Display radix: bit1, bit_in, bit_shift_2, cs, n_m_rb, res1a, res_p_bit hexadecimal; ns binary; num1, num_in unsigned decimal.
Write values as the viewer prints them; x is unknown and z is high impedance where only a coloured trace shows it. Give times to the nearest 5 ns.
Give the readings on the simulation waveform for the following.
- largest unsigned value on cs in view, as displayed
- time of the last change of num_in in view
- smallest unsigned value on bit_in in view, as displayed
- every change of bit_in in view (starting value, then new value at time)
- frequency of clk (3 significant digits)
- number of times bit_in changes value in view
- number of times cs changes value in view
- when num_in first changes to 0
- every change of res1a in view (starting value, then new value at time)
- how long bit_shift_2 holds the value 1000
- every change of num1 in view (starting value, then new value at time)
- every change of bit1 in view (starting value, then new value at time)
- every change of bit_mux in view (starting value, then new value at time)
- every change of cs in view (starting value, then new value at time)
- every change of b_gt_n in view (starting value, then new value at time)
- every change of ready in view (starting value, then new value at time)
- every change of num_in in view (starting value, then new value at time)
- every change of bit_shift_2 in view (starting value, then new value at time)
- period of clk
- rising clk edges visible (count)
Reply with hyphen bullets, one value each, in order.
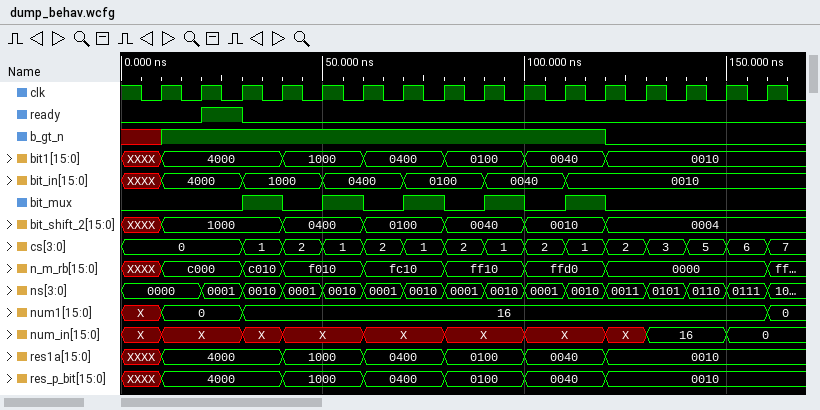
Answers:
- 7
- 150 ns
- 0010
- XXXX, 4000 at 10 ns, 1000 at 30 ns, 0400 at 50 ns, 0100 at 70 ns, 0040 at 90 ns, 0010 at 110 ns
- 100 MHz
- 6
- 14
- 150 ns
- XXXX, 4000 at 10 ns, 1000 at 40 ns, 0400 at 60 ns, 0100 at 80 ns, 0040 at 100 ns, 0010 at 120 ns
- 30 ns
- X, 0 at 10 ns, 16 at 30 ns, 0 at 160 ns
- XXXX, 4000 at 10 ns, 1000 at 40 ns, 0400 at 60 ns, 0100 at 80 ns, 0040 at 100 ns, 0010 at 120 ns
- 0, 1 at 30 ns, 0 at 40 ns, 1 at 50 ns, 0 at 60 ns, 1 at 70 ns, 0 at 80 ns, 1 at 90 ns, 0 at 100 ns, 1 at 110 ns, 0 at 120 ns
- 0, 1 at 30 ns, 2 at 40 ns, 1 at 50 ns, 2 at 60 ns, 1 at 70 ns, 2 at 80 ns, 1 at 90 ns, 2 at 100 ns, 1 at 110 ns, 2 at 120 ns, 3 at 130 ns, 5 at 140 ns, 6 at 150 ns, 7 at 160 ns
- x, 1 at 10 ns, 0 at 120 ns
- 0, 1 at 20 ns, 0 at 30 ns
- X, X at 10 ns, X at 30 ns, X at 40 ns, X at 60 ns, X at 80 ns, X at 100 ns, X at 120 ns, 16 at 130 ns, 0 at 150 ns
- XXXX, 1000 at 10 ns, 0400 at 40 ns, 0100 at 60 ns, 0040 at 80 ns, 0010 at 100 ns, 0004 at 120 ns
- 10 ns
- 16
